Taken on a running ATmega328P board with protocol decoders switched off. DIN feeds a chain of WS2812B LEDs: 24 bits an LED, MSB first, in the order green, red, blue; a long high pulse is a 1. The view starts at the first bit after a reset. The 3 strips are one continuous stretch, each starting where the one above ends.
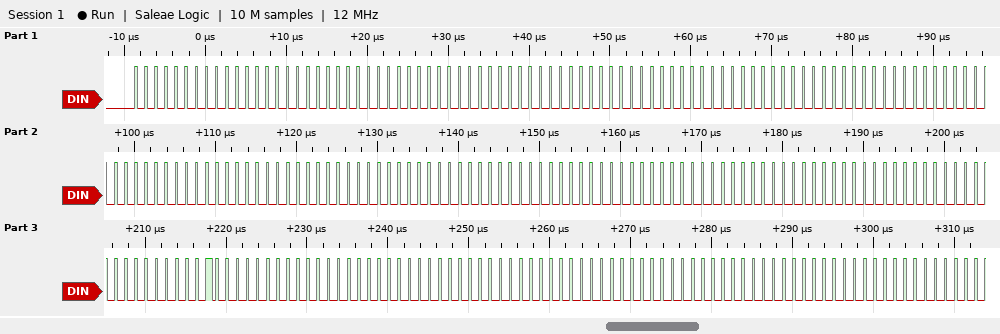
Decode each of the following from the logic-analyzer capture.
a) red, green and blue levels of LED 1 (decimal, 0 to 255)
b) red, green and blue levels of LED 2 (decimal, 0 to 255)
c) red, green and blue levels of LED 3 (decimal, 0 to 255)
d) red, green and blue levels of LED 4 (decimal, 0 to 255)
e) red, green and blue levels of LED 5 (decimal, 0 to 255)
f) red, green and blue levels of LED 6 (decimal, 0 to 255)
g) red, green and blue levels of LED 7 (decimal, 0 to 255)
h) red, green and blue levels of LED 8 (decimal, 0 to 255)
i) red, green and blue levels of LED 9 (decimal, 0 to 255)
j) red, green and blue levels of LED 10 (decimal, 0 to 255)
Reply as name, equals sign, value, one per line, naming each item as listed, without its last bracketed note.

red, green and blue levels of LED 1 = 0, 0, 0
red, green and blue levels of LED 2 = 0, 0, 0
red, green and blue levels of LED 3 = 0, 0, 0
red, green and blue levels of LED 4 = 0, 0, 0
red, green and blue levels of LED 5 = 0, 0, 0
red, green and blue levels of LED 6 = 0, 0, 0
red, green and blue levels of LED 7 = 0, 0, 0
red, green and blue levels of LED 8 = 4, 0, 0
red, green and blue levels of LED 9 = 0, 0, 0
red, green and blue levels of LED 10 = 0, 0, 0
